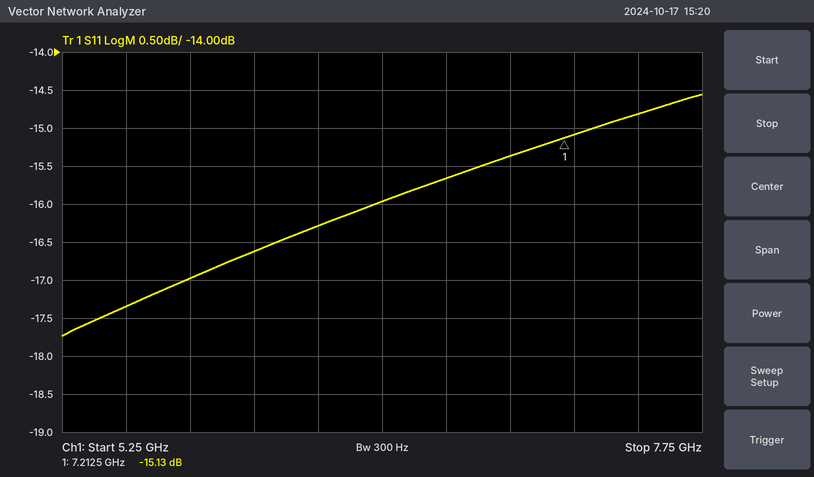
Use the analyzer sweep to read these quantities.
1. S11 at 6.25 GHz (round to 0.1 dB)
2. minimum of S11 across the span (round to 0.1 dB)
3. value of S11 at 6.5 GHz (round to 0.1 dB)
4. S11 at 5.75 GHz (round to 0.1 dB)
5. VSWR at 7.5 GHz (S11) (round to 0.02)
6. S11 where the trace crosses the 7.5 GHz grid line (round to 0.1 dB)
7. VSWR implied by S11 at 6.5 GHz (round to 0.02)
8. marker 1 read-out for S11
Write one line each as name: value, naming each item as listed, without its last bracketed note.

S11 at 6.25 GHz: -16.3 dB
minimum of S11 across the span: -17.7 dB
value of S11 at 6.5 GHz: -16.0 dB
S11 at 5.75 GHz: -17.0 dB
VSWR at 7.5 GHz (S11): 1.44
S11 where the trace crosses the 7.5 GHz grid line: -14.8 dB
VSWR implied by S11 at 6.5 GHz: 1.38
marker 1 read-out for S11: -15.13 dB
